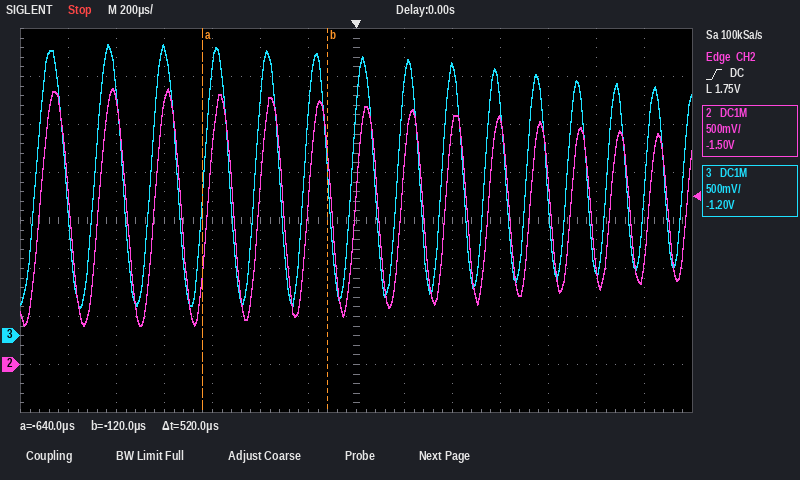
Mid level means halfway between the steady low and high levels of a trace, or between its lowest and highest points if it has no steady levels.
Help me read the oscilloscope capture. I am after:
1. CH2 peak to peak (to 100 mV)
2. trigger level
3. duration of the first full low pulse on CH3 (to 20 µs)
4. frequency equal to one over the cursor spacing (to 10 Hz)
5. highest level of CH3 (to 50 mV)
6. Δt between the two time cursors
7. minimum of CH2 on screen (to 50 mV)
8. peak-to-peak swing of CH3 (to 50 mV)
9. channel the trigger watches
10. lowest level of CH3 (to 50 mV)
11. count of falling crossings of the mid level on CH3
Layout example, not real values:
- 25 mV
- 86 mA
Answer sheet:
- 2.50 V
- 1.75 V
- 120 µs
- 1.92 kHz
- 3.05 V
- 520 µs
- 400 mV
- 2.75 V
- CH2
- 300 mV
- 14
